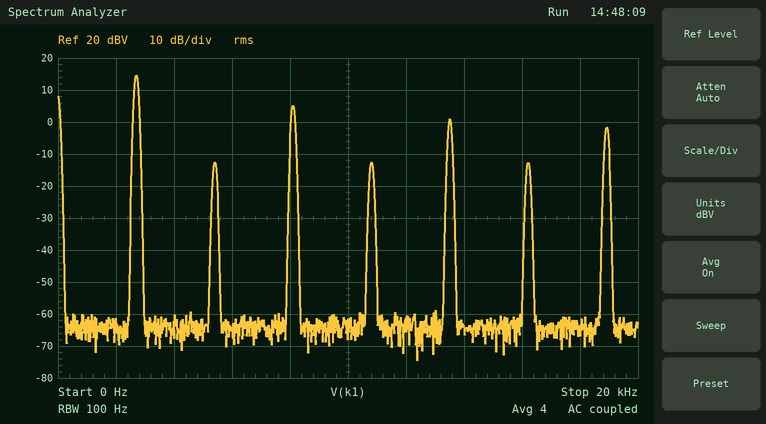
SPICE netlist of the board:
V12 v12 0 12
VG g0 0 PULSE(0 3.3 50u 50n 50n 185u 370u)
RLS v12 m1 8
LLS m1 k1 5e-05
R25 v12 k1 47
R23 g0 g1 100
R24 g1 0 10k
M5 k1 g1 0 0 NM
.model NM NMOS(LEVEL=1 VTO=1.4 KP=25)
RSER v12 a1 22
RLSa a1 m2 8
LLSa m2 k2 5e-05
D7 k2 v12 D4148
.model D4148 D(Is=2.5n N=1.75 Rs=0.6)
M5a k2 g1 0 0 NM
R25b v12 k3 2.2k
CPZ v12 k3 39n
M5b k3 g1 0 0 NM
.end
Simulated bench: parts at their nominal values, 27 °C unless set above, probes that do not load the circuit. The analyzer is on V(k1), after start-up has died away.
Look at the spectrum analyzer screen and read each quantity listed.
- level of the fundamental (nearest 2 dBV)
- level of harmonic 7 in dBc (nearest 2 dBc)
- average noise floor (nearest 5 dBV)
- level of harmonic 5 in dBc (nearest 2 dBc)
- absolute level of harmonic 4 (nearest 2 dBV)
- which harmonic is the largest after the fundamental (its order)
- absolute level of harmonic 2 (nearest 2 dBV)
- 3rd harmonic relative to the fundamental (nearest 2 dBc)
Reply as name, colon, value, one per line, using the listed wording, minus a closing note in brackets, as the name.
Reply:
level of the fundamental: 14 dBV
level of harmonic 7 in dBc: -16 dBc
average noise floor: -65 dBV
level of harmonic 5 in dBc: -14 dBc
absolute level of harmonic 4: -12 dBV
which harmonic is the largest after the fundamental: 3
absolute level of harmonic 2: -12 dBV
3rd harmonic relative to the fundamental: -10 dBc
